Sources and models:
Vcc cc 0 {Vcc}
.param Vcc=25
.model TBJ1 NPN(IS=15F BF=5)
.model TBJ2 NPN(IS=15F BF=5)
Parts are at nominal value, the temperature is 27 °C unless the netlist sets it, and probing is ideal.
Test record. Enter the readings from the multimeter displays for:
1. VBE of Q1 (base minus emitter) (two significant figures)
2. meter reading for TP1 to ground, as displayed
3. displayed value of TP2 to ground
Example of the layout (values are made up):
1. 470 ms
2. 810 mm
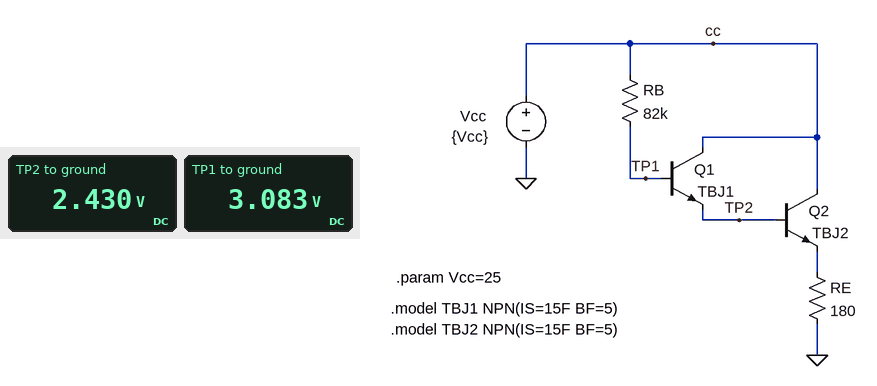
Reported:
1. 650 mV
2. 3.083 V
3. 2.430 V
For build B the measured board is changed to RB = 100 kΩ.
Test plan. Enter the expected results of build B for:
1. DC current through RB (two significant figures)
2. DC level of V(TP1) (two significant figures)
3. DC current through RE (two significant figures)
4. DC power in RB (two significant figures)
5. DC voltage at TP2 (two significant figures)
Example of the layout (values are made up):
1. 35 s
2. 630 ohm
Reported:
1. 220 µA
2. 2.8 V
3. 8.0 mA
4. 4.9 mW
5. 2.1 V
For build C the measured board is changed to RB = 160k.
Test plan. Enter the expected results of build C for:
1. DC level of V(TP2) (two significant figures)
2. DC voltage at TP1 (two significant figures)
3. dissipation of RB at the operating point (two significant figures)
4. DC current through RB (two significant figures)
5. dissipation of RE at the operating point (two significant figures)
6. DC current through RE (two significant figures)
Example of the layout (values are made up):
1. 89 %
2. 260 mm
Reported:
1. 1.6 V
2. 2.2 V
3. 3.2 mW
4. 140 µA
5. 4.7 mW
6. 5.1 mA
